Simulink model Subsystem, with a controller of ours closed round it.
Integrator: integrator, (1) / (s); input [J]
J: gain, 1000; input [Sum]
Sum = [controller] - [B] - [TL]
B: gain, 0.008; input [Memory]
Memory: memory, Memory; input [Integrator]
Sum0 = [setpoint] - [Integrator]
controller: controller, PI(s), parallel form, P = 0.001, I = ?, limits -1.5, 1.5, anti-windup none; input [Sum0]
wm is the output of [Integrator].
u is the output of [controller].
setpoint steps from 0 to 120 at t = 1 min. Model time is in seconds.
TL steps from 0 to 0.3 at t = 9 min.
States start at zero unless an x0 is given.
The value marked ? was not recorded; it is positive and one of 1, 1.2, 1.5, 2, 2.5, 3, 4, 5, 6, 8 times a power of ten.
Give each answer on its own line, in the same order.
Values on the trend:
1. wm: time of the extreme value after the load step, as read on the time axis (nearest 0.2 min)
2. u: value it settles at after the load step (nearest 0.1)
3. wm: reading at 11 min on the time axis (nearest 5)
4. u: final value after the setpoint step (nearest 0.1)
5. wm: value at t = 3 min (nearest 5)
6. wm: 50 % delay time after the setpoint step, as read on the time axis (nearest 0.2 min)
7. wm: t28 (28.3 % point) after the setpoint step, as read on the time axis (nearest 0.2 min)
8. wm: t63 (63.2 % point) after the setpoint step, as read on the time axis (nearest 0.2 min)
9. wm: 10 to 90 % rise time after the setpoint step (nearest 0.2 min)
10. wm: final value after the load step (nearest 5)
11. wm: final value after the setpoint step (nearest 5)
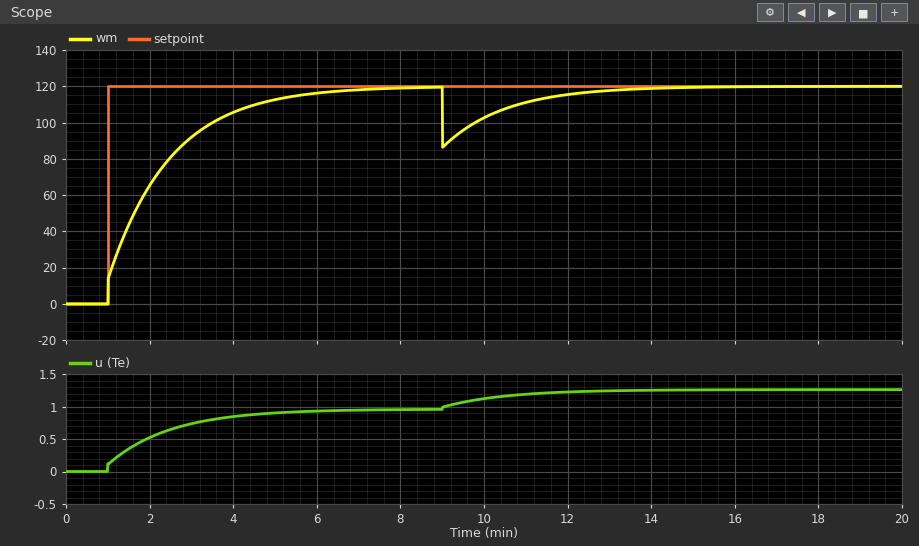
9.0 min
1.3
110
1.0
90
1.8 min
1.4 min
2.4 min
3.2 min
120
120
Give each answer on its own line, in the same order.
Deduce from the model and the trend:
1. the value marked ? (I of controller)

0.0001
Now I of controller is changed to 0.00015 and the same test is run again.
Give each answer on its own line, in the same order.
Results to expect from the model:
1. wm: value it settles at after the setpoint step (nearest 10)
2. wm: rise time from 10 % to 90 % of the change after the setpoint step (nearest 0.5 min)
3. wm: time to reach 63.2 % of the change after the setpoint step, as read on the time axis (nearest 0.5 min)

120
2.0 min
2.0 min
